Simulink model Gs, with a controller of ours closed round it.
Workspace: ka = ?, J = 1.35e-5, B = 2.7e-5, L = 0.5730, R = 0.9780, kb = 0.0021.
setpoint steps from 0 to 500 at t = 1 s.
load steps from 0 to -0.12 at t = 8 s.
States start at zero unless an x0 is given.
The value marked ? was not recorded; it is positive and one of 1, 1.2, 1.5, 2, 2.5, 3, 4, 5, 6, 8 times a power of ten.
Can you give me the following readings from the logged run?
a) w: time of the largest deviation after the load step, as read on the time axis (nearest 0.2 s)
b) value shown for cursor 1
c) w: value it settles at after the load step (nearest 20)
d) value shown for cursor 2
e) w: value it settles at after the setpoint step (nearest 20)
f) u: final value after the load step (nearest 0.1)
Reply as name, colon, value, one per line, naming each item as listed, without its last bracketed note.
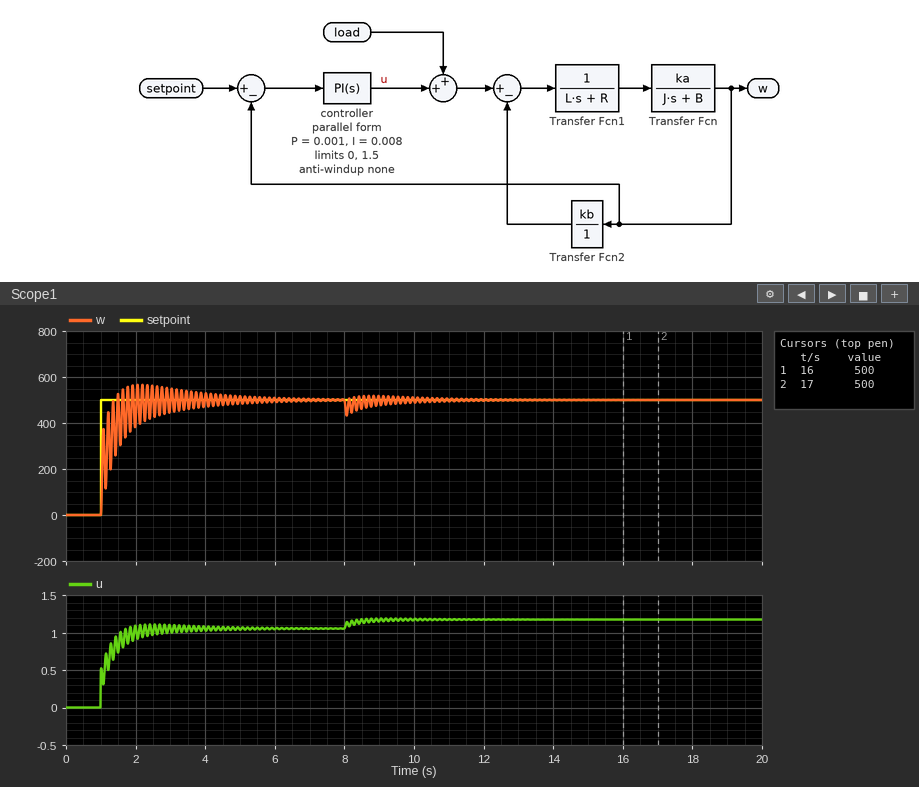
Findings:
w: time of the largest deviation after the load step, as read on the time axis: 8.0 s
value shown for cursor 1: 500
w: value it settles at after the load step: 500
value shown for cursor 2: 500
w: value it settles at after the setpoint step: 500
u: final value after the load step: 1.2
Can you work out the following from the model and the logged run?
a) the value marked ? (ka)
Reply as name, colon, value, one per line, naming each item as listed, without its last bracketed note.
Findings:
the value marked ?: 5
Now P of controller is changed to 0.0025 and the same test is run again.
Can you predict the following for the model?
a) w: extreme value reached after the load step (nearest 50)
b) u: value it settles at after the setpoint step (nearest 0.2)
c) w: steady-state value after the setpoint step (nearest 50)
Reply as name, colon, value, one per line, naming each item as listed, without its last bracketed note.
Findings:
w: extreme value reached after the load step: 450
u: value it settles at after the setpoint step: 1.0
w: steady-state value after the setpoint step: 500
